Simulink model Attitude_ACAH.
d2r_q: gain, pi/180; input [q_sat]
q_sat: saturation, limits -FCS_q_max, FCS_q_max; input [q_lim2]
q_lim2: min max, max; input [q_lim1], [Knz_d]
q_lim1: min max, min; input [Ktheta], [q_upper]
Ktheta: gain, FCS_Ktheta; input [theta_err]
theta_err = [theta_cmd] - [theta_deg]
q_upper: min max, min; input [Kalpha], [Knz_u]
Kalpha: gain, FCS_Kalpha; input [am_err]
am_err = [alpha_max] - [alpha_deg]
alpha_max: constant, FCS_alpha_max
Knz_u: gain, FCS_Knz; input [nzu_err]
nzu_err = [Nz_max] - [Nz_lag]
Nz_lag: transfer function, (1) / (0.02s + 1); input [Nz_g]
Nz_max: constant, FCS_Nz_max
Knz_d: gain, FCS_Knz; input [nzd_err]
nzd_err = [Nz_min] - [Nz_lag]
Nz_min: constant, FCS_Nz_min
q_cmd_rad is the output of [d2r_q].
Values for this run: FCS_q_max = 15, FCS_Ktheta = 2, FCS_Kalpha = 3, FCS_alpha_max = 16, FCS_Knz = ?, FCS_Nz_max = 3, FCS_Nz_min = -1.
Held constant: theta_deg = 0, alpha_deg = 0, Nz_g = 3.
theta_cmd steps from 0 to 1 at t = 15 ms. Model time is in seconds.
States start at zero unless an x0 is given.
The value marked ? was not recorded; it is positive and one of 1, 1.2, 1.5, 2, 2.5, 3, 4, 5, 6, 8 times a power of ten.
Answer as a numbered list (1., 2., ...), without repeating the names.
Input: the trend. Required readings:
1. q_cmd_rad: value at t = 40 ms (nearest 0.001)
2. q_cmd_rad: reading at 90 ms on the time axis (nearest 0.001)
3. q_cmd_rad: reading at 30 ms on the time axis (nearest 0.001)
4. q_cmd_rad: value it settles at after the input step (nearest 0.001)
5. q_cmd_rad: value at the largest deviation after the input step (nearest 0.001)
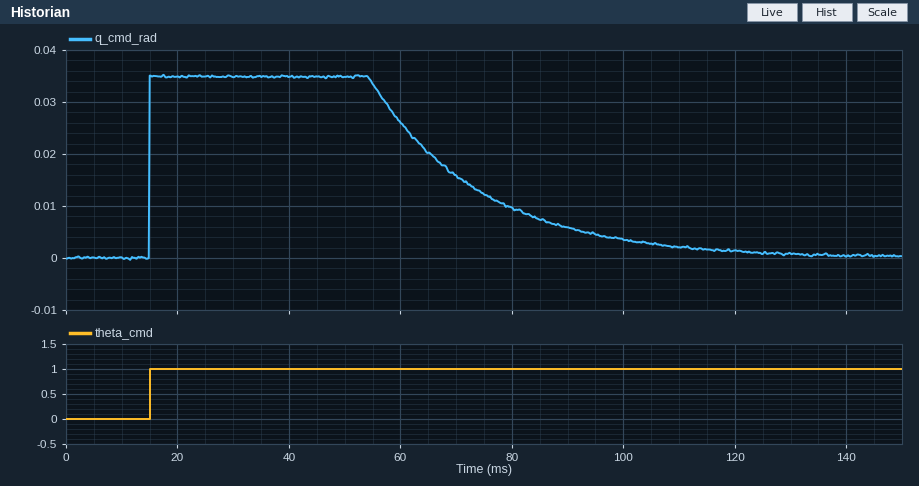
1. 0.035
2. 0.006
3. 0.035
4. 0.000
5. 0.035
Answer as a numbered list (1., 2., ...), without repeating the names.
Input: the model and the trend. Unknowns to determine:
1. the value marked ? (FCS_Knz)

1. 10
